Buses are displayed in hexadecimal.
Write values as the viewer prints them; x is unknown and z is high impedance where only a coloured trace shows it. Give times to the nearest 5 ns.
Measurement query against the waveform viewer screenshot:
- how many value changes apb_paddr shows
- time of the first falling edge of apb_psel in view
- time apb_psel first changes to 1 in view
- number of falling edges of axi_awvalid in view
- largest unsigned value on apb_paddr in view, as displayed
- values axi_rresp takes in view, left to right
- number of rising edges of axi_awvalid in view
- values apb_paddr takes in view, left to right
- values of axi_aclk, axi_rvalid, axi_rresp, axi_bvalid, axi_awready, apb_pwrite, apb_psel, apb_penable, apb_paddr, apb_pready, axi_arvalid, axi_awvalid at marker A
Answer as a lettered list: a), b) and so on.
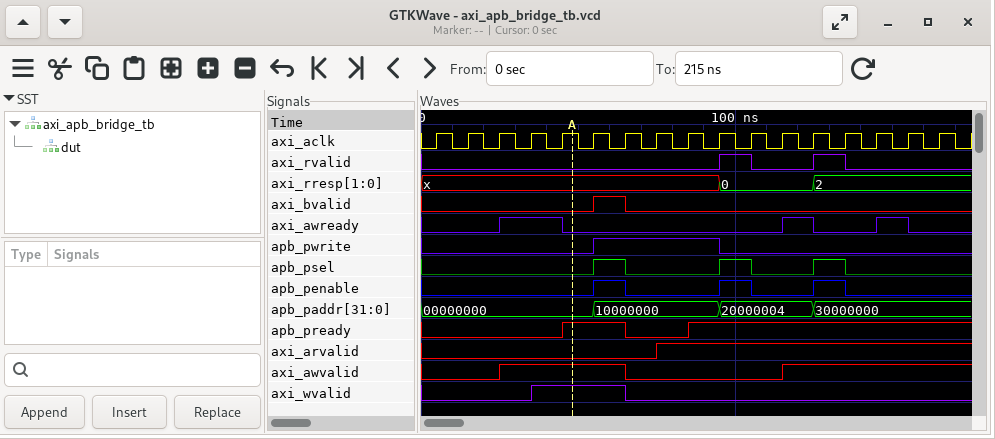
a) 3
b) 65 ns
c) 55 ns
d) 1
e) 30000000
f) x, 0, 2
g) 2
h) 00000000, 10000000, 20000004, 30000000
i) axi_aclk=1, axi_rvalid=0, axi_rresp=x, axi_bvalid=0, axi_awready=0, apb_pwrite=0, apb_psel=0, apb_penable=0, apb_paddr=00000000, apb_pready=1, axi_arvalid=0, axi_awvalid=1
